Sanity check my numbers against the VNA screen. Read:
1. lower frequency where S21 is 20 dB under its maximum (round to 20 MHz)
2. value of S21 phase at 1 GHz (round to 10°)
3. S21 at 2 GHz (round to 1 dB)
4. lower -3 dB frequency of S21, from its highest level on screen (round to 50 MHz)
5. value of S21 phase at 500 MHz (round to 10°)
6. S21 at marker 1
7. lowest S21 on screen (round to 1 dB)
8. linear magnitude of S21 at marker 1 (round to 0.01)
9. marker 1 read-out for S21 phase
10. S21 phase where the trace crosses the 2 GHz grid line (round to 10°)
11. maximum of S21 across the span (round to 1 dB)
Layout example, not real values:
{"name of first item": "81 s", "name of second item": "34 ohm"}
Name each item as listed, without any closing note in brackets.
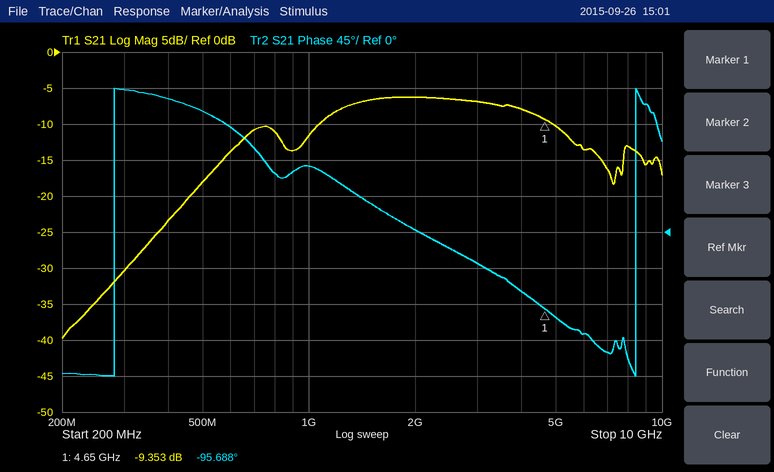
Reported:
{"lower frequency where S21 is 20 dB under its maximum": "360 MHz", "value of S21 phase at 1 GHz": "80°", "S21 at 2 GHz": "-6 dB", "lower -3 dB frequency of S21, from its highest level on screen": "1.10 GHz", "value of S21 phase at 500 MHz": "150°", "S21 at marker 1": "-9.353 dB", "lowest S21 on screen": "-40 dB", "linear magnitude of S21 at marker 1": "0.34", "marker 1 read-out for S21 phase": "-95.688°", "S21 phase where the trace crosses the 2 GHz grid line": "0°", "maximum of S21 across the span": "-6 dB"}
